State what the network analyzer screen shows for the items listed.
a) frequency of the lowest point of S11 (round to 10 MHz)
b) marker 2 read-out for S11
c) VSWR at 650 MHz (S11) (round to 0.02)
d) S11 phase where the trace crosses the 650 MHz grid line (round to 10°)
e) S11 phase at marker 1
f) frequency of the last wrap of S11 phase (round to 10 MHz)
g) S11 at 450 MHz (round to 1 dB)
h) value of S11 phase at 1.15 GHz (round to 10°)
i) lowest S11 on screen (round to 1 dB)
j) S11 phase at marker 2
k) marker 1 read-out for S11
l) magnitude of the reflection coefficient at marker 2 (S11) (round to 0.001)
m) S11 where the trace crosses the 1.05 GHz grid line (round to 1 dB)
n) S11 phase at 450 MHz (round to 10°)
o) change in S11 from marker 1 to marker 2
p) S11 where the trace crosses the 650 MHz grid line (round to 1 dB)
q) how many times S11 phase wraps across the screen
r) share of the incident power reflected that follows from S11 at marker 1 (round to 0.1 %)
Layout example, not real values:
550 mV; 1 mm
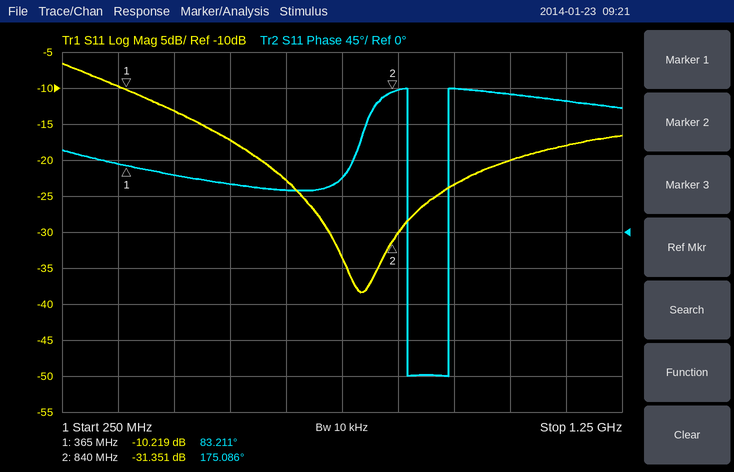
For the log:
780 MHz; -31.351 dB; 1.16; 50°; 83.211°; 940 MHz; -13 dB; 160°; -38 dB; 175.086°; -10.219 dB; 0.027; -20 dB; 70°; -21.132 dB; -23 dB; 2; 9.5 %
